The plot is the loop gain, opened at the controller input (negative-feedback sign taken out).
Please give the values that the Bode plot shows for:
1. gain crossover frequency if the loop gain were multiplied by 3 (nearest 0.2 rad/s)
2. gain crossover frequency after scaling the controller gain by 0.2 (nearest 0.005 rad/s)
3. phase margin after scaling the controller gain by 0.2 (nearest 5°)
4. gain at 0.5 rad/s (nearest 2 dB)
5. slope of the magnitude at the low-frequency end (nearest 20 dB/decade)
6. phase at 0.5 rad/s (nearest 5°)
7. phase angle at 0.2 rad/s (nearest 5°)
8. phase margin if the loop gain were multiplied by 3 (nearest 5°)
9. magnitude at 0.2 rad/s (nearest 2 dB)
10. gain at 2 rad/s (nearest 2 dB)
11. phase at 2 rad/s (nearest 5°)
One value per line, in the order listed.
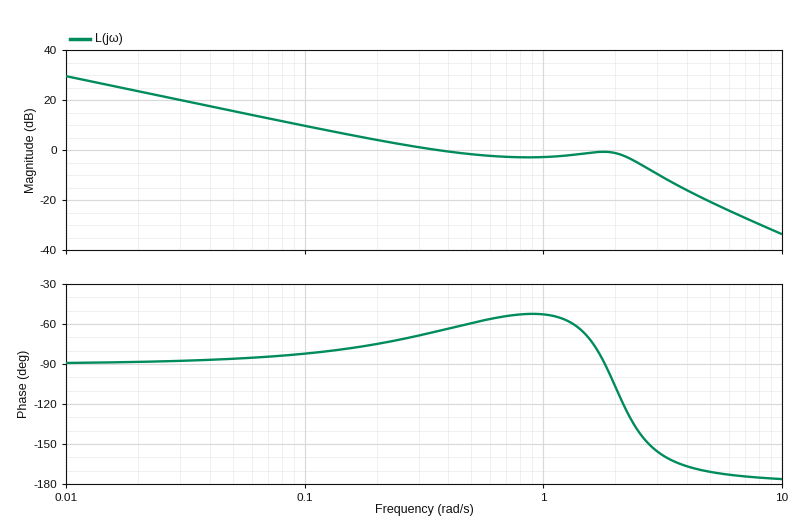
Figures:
3.0 rad/s
0.060 rad/s
95°
-2 dB
-20 dB/decade
-60°
-75°
25°
4 dB
-2 dB
-105°
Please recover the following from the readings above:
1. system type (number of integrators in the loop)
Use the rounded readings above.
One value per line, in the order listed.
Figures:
1
